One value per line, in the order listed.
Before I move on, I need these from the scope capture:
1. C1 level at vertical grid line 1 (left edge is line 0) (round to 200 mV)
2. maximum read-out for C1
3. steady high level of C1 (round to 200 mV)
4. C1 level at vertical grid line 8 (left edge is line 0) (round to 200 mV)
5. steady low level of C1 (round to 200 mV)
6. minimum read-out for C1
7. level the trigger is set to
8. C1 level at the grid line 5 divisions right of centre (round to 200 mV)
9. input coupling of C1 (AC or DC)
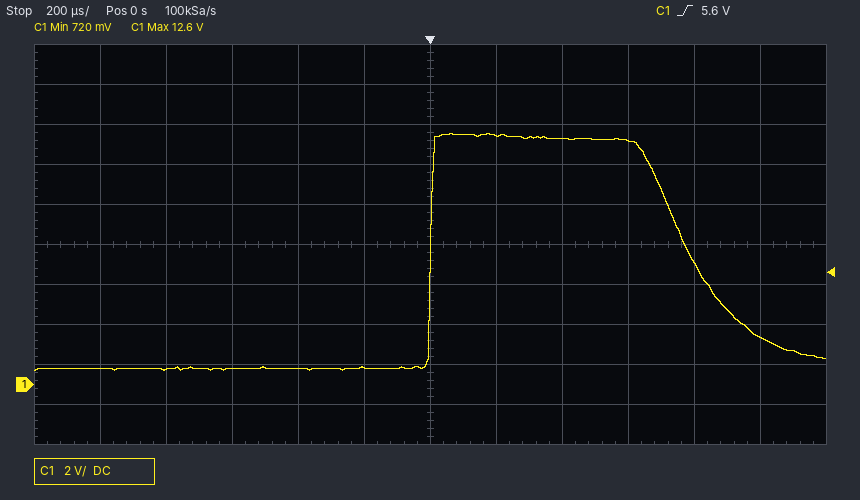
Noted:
800 mV
12.6 V
12.4 V
12.4 V
800 mV
720 mV
5.6 V
2.4 V
DC
